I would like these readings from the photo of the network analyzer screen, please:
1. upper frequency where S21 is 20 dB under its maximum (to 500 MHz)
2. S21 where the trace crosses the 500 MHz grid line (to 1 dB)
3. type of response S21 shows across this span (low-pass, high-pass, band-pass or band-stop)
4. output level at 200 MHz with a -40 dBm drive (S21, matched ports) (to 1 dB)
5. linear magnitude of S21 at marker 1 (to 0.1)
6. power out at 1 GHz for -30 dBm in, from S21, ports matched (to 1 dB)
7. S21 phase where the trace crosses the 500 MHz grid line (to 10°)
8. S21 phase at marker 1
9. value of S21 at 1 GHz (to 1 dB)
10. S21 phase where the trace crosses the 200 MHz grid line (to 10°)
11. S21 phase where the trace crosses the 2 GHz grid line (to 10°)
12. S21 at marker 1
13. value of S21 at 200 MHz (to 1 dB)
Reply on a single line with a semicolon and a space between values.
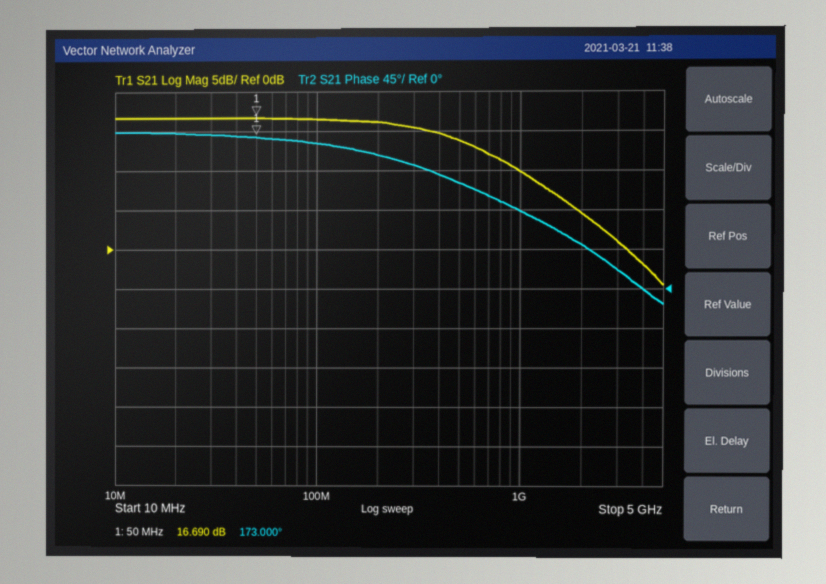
4.5 GHz; 14 dB; low-pass; -24 dBm; 6.8; -20 dBm; 120°; 173.000°; 10 dB; 150°; 50°; 16.690 dB; 16 dB
